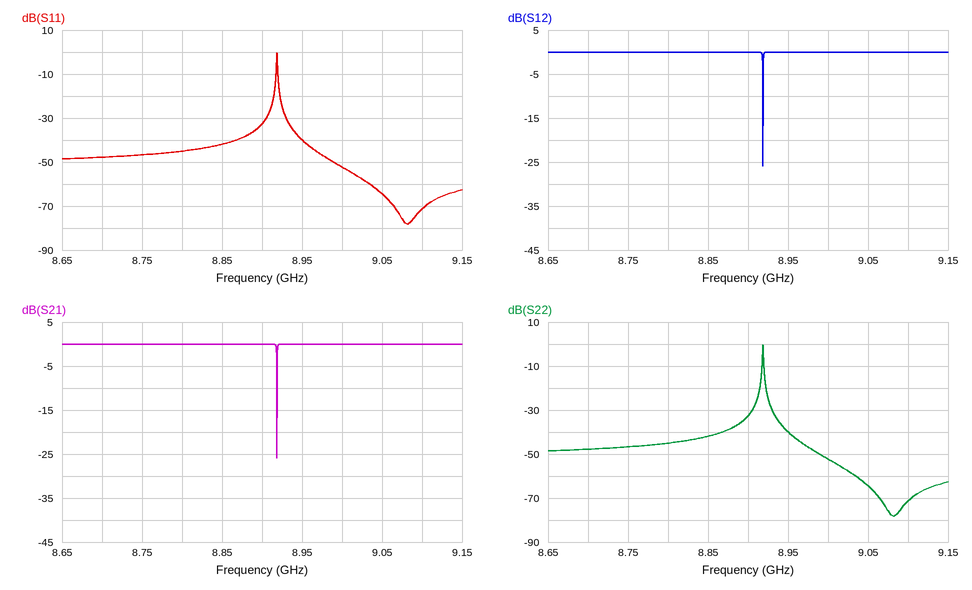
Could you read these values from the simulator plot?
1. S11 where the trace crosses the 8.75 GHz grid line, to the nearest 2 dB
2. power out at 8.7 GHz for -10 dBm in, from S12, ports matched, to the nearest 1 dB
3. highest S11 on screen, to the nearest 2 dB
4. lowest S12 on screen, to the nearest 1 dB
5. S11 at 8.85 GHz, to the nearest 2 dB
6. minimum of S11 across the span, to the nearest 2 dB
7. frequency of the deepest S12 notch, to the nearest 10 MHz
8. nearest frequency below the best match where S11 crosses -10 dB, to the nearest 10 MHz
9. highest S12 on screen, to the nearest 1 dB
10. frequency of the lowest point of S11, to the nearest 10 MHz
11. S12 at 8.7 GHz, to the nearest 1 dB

-46 dB
-10 dBm
0 dB
-26 dB
-42 dB
-78 dB
8.92 GHz
8.92 GHz
0 dB
9.08 GHz
0 dB
